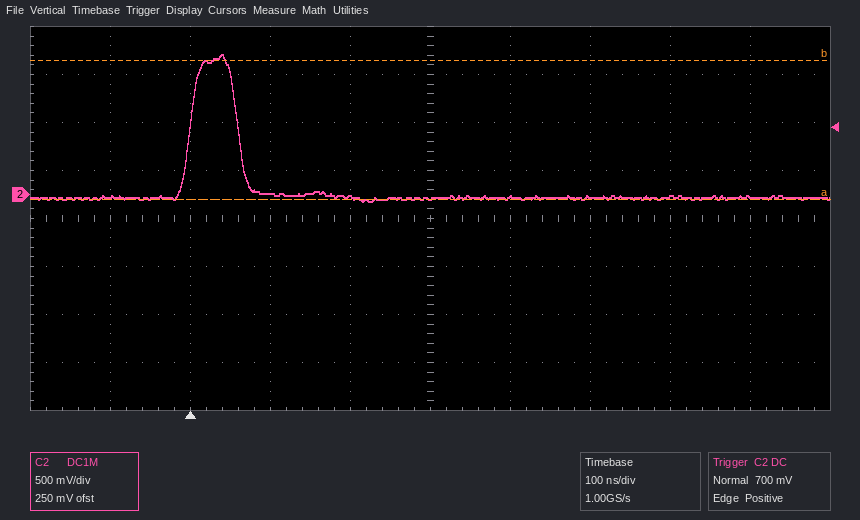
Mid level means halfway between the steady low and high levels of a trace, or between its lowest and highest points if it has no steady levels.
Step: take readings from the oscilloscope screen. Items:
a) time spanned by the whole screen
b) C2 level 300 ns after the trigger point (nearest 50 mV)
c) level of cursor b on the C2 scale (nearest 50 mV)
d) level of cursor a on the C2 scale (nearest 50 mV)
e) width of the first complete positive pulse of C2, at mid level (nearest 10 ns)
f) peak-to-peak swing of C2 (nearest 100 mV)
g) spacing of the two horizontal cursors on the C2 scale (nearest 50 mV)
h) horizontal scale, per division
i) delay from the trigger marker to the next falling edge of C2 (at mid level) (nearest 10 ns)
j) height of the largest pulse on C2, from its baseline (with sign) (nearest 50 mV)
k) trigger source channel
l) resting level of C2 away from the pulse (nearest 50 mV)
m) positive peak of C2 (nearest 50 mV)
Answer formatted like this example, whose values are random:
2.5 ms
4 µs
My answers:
1 µs
-50 mV
1.40 V
-50 mV
60 ns
1.50 V
1.45 V
100 ns
60 ns
+1.50 V
C2
-50 mV
1.45 V
